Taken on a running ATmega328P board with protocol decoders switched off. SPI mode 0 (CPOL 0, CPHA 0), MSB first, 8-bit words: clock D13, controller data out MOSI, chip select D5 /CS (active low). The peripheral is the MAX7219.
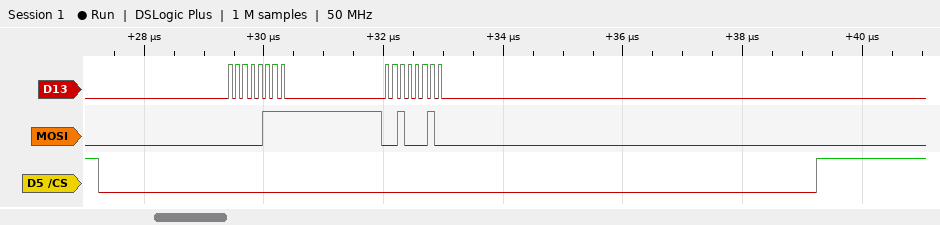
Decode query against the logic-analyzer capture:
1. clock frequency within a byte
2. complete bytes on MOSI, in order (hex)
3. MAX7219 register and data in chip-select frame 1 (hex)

8 MHz
0x07 0x22
register 0x7, data 0x22
